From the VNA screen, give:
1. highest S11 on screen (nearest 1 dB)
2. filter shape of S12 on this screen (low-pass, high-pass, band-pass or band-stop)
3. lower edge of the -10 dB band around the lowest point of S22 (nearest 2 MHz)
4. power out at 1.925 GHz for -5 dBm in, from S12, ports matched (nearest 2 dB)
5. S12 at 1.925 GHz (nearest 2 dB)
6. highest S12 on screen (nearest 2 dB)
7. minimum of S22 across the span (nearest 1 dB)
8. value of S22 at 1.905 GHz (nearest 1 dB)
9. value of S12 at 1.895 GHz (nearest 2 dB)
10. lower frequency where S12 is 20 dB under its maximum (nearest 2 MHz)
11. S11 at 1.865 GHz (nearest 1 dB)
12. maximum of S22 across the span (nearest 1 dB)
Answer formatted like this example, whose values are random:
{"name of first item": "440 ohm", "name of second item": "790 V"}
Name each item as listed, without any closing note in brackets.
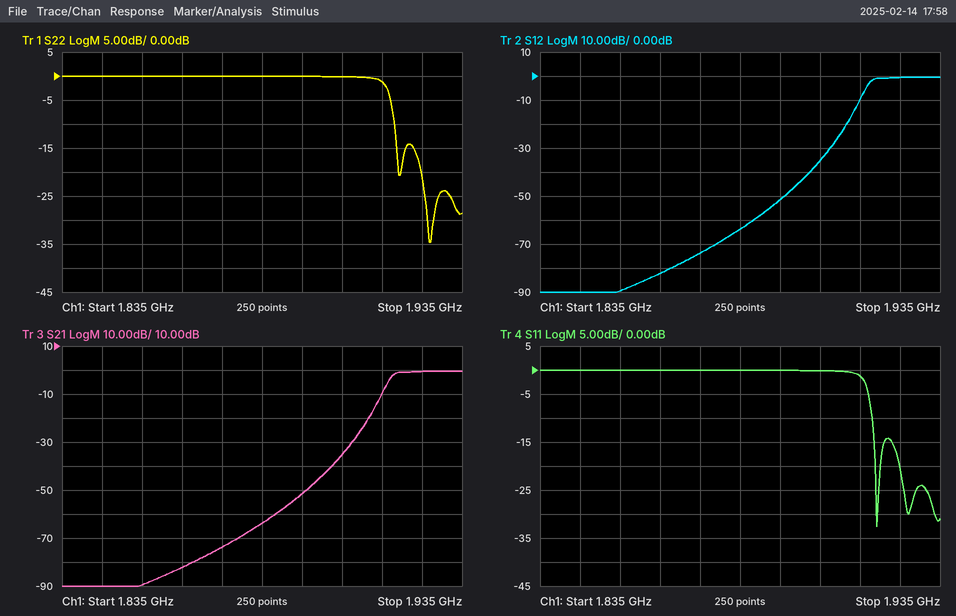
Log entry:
{"highest S11 on screen": "0 dB", "filter shape of S12 on this screen": "high-pass", "lower edge of the -10 dB band around the lowest point of S22": "1.918 GHz", "power out at 1.925 GHz for -5 dBm in, from S12, ports matched": "-6 dBm", "S12 at 1.925 GHz": "0 dB", "highest S12 on screen": "0 dB", "minimum of S22 across the span": "-35 dB", "value of S22 at 1.905 GHz": "0 dB", "value of S12 at 1.895 GHz": "-52 dB", "lower frequency where S12 is 20 dB under its maximum": "1.912 GHz", "S11 at 1.865 GHz": "0 dB", "maximum of S22 across the span": "0 dB"}
